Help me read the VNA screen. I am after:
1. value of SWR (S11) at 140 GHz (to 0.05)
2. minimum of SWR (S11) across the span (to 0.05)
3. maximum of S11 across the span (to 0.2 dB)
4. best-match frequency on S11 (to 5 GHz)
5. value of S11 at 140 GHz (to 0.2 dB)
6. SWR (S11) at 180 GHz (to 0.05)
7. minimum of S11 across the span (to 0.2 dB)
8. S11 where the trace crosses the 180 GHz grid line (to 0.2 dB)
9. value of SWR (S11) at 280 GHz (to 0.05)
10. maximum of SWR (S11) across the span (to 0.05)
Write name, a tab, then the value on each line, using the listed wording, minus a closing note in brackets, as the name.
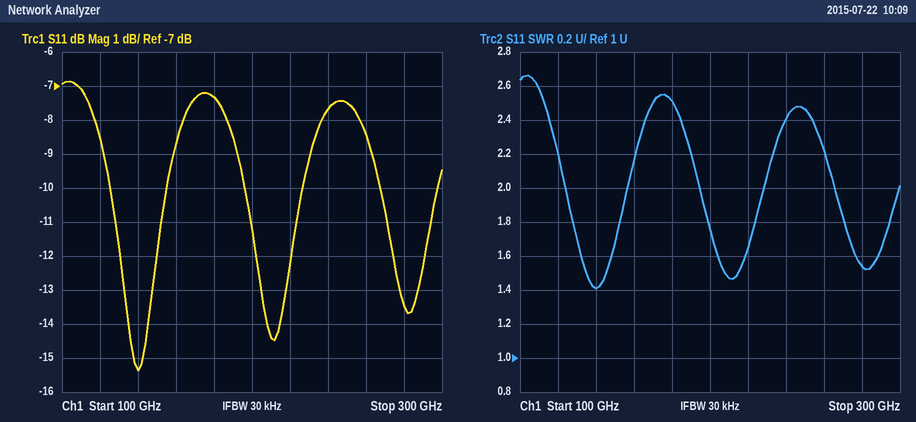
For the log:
value of SWR (S11) at 140 GHz	1.40
minimum of SWR (S11) across the span	1.40
maximum of S11 across the span	-6.8 dB
best-match frequency on S11	140 GHz
value of S11 at 140 GHz	-15.4 dB
SWR (S11) at 180 GHz	2.50
minimum of S11 across the span	-15.4 dB
S11 where the trace crosses the 180 GHz grid line	-7.4 dB
value of SWR (S11) at 280 GHz	1.55
maximum of SWR (S11) across the span	2.65
